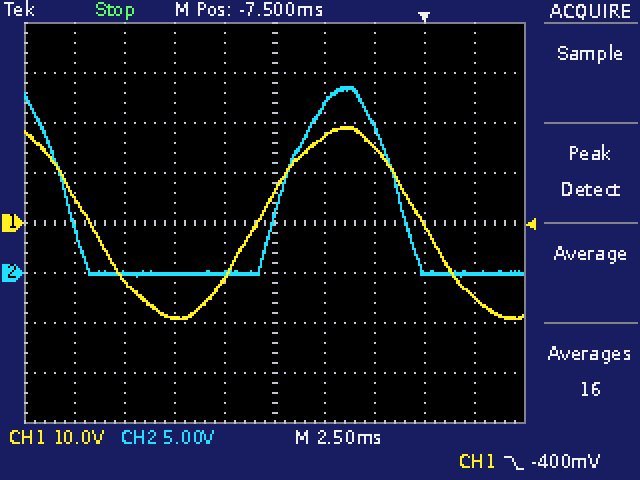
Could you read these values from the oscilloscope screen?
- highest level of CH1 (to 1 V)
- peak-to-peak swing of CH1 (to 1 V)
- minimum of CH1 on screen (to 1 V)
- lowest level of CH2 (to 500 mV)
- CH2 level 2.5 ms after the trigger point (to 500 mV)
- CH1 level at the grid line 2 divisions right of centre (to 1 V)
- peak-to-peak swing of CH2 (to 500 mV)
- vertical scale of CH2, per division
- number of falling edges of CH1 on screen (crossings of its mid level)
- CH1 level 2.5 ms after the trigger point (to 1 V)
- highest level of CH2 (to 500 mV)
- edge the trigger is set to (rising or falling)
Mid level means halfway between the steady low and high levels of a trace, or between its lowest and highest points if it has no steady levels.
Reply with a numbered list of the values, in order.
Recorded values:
1. 19 V
2. 38 V
3. -19 V
4. -500 mV
5. 0.0 V
6. 15 V
7. 19.0 V
8. 5 V
9. 2
10. -15 V
11. 18.5 V
12. falling
